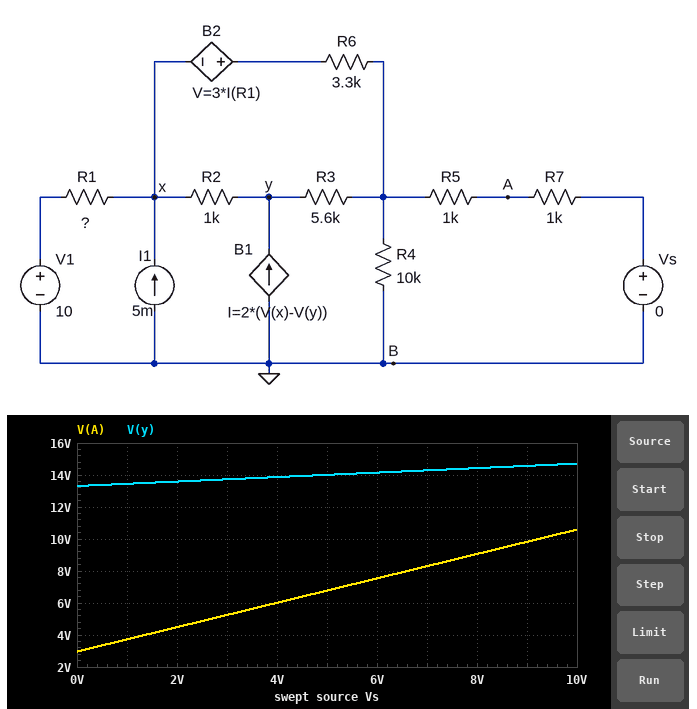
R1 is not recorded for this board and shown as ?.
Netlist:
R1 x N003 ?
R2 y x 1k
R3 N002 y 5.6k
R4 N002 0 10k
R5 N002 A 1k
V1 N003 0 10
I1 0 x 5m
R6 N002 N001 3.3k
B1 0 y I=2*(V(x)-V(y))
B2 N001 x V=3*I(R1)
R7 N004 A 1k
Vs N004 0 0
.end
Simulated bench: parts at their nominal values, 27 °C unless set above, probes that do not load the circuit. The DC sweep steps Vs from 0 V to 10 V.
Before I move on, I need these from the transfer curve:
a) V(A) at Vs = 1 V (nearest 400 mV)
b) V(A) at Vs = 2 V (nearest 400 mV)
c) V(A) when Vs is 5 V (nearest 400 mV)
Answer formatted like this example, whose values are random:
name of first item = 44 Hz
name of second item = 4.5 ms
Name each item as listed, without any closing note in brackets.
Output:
V(A) at Vs = 1 V = 3.6 V
V(A) at Vs = 2 V = 4.4 V
V(A) when Vs is 5 V = 6.8 V
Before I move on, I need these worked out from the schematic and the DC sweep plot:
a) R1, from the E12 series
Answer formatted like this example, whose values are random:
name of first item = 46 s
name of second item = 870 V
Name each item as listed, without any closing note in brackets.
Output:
R1, from the E12 series = 1.2 kΩ
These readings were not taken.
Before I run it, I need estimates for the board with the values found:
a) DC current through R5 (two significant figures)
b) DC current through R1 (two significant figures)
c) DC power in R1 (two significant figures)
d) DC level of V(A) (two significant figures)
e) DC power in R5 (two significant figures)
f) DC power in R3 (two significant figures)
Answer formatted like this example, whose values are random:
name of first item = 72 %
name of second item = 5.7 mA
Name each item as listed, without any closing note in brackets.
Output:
DC current through R5 = 3.0 mA
DC current through R1 = 2.8 mA
DC power in R1 = 9.1 mW
DC level of V(A) = 3.0 V
DC power in R5 = 8.8 mW
DC power in R3 = 9.7 mW
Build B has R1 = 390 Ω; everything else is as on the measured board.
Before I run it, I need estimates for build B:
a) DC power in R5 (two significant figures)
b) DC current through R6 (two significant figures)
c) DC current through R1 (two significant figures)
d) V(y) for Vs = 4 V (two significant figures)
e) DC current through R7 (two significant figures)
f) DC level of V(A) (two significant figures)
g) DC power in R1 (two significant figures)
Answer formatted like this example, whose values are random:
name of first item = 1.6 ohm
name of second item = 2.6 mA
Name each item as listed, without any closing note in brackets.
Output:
DC power in R5 = 6.2 mW
DC current through R6 = 1.9 mA
DC current through R1 = 3.1 mA
V(y) for Vs = 4 V = 11 V
DC current through R7 = 2.5 mA
DC level of V(A) = 2.5 V
DC power in R1 = 3.8 mW
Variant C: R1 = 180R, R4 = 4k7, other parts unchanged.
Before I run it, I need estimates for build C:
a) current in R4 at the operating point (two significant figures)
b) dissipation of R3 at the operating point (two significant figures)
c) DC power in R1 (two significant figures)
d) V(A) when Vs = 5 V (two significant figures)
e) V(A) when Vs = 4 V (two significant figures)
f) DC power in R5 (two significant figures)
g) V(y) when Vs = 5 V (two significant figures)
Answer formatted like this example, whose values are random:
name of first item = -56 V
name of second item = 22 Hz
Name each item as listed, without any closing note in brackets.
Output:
current in R4 at the operating point = 910 µA
dissipation of R3 at the operating point = 7.1 mW
DC power in R1 = 1.7 mW
V(A) when Vs = 5 V = 5.7 V
V(A) when Vs = 4 V = 5.0 V
DC power in R5 = 4.5 mW
V(y) when Vs = 5 V = 11 V
